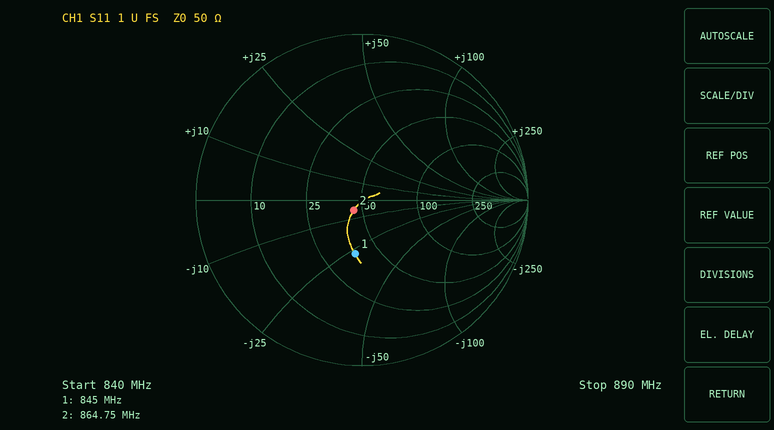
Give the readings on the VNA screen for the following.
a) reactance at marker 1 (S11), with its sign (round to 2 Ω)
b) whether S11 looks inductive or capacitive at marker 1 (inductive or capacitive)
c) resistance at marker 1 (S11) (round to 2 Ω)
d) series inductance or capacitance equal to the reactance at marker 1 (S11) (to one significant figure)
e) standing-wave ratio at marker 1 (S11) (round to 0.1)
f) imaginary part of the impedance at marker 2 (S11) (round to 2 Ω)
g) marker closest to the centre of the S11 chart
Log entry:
-28 Ω
capacitive
38 Ω
7 pF
2.0
-6 Ω
marker 2
